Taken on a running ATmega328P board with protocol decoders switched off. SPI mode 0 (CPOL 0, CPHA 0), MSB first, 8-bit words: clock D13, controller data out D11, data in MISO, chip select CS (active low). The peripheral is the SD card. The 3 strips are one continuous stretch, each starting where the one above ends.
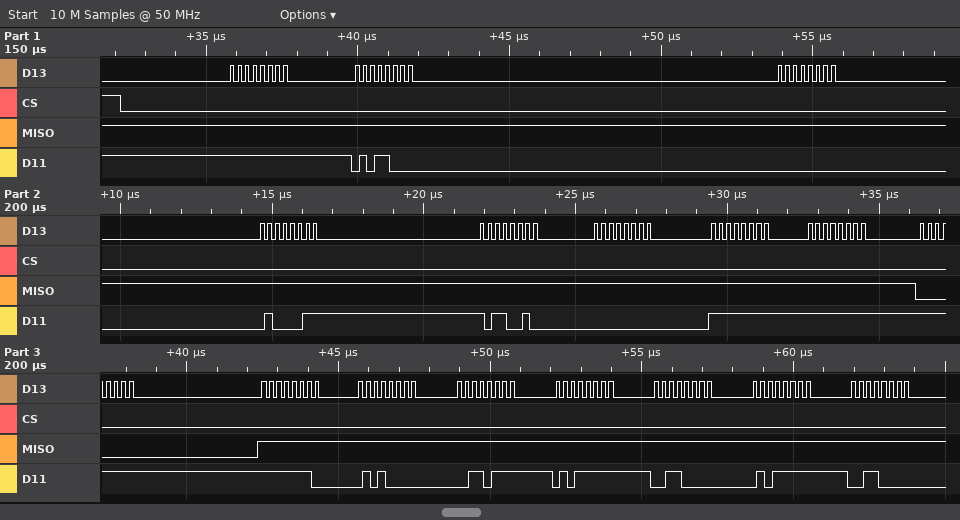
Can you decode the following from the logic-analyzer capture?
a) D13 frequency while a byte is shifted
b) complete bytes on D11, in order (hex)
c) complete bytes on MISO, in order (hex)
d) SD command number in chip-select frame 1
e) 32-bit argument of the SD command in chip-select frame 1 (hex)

4 MHz
0xFF 0x58 0x00 0x43 0xB2 0x00 0xFF 0xFF 0xFF 0xFE 0x50 0x37 0x5F 0x30 0x5F 0x30
0xFF 0xFF 0xFF 0xFF 0xFF 0xFF 0xFF 0xFF 0x00 0xFF 0xFF 0xFF 0xFF 0xFF 0xFF 0xFF
CMD24
0x0043B200
